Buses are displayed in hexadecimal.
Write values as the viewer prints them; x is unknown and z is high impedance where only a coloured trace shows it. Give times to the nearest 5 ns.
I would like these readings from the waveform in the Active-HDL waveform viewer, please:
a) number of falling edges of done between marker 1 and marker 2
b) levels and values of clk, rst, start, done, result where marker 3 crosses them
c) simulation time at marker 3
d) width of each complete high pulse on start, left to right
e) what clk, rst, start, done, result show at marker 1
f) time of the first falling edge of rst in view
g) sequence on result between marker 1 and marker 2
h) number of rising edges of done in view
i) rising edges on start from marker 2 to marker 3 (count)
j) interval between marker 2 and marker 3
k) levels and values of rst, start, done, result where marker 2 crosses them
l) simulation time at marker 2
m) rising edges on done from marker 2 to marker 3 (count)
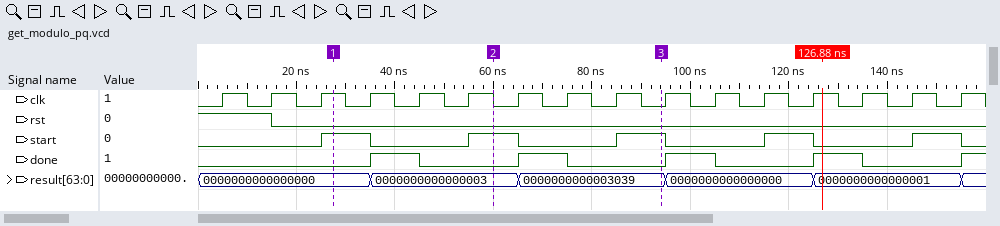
1
clk=0, rst=0, start=1, done=0, result=0000000000003039
95 ns
10 ns, 10 ns, 10 ns, 10 ns, 10 ns
clk=1, rst=0, start=1, done=0, result=0000000000000000
15 ns
0000000000000000, 0000000000000003
5
1
35 ns
rst=0, start=1, done=0, result=0000000000000003
60 ns
1
